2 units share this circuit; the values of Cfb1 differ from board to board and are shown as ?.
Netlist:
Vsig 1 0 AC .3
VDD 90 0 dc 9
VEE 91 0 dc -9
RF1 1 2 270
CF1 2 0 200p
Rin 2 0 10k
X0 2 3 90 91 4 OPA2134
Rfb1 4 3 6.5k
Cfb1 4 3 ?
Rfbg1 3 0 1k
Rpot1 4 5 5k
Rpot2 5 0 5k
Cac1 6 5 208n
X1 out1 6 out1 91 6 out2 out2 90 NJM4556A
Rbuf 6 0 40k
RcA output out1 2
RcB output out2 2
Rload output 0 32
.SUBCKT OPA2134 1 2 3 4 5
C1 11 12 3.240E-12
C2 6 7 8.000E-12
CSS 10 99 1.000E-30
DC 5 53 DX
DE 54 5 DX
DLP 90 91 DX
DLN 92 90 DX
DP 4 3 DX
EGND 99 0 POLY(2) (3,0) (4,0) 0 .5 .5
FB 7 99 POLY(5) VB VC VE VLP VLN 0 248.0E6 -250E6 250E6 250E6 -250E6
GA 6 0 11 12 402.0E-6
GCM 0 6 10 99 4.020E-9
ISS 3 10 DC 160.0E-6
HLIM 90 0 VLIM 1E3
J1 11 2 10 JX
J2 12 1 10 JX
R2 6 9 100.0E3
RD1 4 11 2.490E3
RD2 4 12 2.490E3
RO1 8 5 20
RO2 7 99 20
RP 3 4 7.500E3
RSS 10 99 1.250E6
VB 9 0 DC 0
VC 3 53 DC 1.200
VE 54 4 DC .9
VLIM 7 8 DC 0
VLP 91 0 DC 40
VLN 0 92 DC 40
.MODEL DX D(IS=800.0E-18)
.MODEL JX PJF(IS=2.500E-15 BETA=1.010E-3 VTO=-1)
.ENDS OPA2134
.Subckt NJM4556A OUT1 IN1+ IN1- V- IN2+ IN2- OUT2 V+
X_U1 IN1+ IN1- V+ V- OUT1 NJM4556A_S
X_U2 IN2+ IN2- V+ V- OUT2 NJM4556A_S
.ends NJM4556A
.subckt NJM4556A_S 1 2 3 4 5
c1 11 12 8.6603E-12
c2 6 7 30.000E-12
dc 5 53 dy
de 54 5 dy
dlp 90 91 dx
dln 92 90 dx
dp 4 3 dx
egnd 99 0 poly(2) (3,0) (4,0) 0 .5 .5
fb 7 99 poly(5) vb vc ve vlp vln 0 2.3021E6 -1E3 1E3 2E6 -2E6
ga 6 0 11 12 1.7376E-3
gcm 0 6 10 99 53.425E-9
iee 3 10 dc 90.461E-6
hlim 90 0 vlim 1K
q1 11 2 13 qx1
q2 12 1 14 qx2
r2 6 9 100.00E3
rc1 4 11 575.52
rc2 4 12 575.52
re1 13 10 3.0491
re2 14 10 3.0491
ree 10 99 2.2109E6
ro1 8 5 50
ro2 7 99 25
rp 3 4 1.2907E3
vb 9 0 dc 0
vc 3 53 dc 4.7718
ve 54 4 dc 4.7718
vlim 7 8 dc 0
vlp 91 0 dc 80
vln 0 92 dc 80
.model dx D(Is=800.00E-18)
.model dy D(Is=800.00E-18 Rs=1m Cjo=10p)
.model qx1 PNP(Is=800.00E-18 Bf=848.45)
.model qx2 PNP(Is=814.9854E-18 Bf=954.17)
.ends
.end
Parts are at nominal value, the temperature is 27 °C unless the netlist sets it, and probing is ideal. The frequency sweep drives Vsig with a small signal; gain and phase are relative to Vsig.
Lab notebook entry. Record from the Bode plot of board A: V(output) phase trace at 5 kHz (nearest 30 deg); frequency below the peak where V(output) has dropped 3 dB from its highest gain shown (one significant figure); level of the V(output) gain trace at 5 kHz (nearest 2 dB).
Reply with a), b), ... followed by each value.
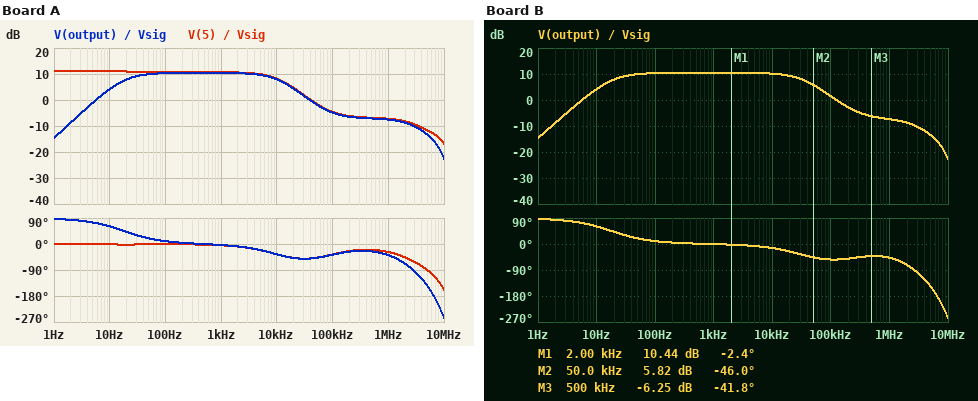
a) -30 deg
b) 20 Hz
c) 10 dB
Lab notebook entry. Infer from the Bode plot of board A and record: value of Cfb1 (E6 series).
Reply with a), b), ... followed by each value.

a) 2.2 nF
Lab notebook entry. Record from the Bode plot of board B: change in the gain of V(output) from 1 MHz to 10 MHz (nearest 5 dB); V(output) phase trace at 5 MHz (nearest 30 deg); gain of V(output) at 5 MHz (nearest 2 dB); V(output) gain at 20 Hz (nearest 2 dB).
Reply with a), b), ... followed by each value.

a) -15 dB
b) -150 deg
c) -14 dB
d) 8 dB
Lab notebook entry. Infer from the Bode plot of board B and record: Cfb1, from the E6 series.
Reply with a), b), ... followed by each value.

a) 680 pF
